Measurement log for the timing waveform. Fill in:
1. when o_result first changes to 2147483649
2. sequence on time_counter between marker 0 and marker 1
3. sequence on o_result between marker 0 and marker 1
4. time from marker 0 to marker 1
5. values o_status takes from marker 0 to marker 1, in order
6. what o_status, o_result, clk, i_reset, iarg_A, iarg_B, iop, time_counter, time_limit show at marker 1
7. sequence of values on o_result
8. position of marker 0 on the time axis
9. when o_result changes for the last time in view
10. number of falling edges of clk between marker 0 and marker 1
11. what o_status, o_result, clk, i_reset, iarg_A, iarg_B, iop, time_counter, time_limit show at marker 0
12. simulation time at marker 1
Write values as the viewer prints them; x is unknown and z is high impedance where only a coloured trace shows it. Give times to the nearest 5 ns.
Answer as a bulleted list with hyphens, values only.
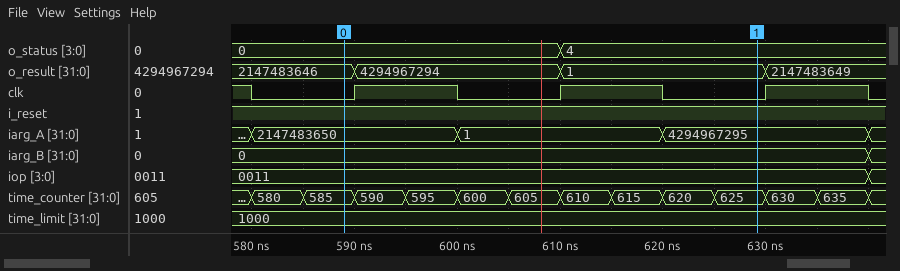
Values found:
- 630 ns
- 585, 590, 595, 600, 605, 610, 615, 620, 625
- 2147483646, 4294967294, 1
- 40 ns
- 0, 4
- o_status=4, o_result=1, clk=0, i_reset=1, iarg_A=4294967295, iarg_B=0, iop=0011, time_counter=625, time_limit=1000
- 2147483646, 4294967294, 1, 2147483649
- 590 ns
- 630 ns
- 2
- o_status=0, o_result=2147483646, clk=0, i_reset=1, iarg_A=2147483650, iarg_B=0, iop=0011, time_counter=585, time_limit=1000
- 630 ns
